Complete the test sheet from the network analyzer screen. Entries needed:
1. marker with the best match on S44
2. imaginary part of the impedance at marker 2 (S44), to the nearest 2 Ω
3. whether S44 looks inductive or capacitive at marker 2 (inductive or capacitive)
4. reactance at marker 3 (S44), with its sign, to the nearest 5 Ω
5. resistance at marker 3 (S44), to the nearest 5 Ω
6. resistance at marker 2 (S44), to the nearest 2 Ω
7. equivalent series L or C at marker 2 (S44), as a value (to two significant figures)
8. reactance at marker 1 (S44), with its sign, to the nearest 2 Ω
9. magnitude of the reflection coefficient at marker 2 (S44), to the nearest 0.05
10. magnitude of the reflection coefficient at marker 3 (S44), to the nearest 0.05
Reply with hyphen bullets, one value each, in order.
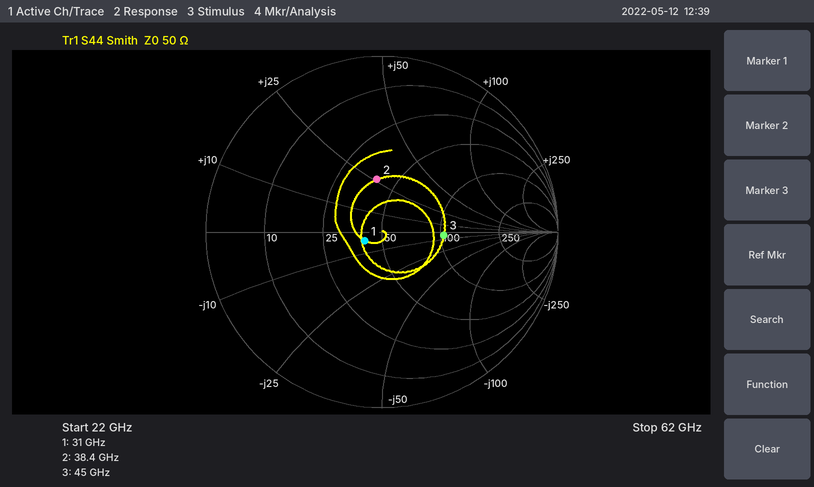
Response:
- marker 1
- +26 Ω
- inductive
- -5 Ω
- 105 Ω
- 40 Ω
- 110 pH
- -4 Ω
- 0.30
- 0.35
